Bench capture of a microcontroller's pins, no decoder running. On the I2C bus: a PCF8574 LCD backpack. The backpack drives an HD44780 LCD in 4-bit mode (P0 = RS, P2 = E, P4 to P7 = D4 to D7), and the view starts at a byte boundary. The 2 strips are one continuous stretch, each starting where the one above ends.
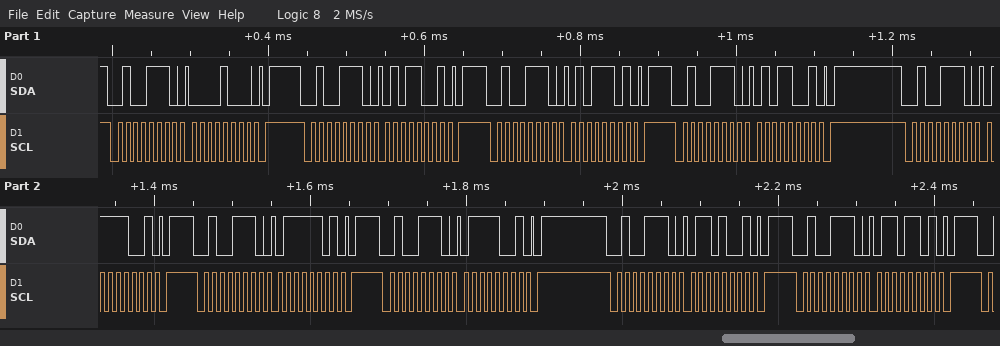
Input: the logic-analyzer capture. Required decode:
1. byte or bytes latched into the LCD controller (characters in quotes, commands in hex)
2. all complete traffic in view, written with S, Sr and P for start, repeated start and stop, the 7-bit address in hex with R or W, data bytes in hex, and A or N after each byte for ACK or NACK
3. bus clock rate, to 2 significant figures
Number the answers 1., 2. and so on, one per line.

1. 'W'
2. S 27W A 08 A P S 27W A 59 A P S 27W A 5D A P S 27W A 59 A P S 27W A 79 A P S 27W A 7D A P S 27W A 79 A P S 27W A 69 A P S 27W A 6D A P
3. 100 kHz
